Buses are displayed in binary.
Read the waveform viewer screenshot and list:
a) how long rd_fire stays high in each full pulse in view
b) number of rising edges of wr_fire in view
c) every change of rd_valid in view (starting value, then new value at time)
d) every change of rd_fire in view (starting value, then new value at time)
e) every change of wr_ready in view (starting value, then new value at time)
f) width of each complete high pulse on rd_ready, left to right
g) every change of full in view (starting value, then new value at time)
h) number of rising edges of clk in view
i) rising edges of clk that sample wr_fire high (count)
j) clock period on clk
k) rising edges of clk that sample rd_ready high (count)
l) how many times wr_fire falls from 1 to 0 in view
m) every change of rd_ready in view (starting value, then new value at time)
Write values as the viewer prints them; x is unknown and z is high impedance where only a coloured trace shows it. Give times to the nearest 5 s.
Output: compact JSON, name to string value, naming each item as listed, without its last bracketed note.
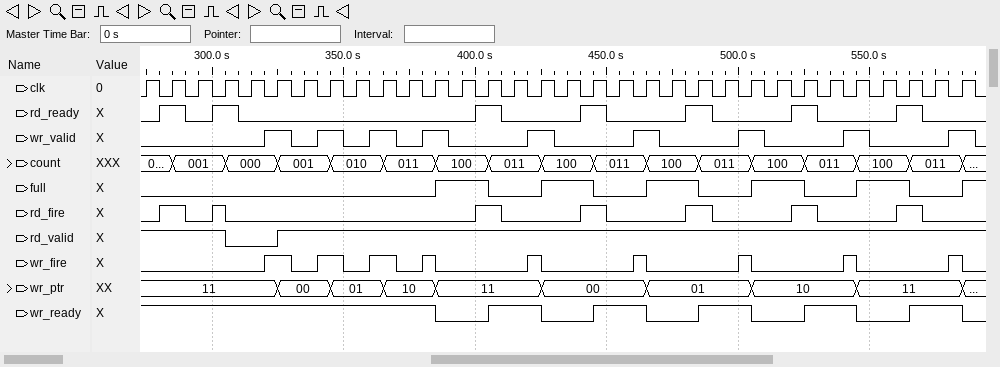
{"how long rd_fire stays high in each full pulse in view": "10 s, 5 s, 10 s, 10 s, 10 s, 10 s, 10 s", "number of rising edges of wr_fire in view": "9", "every change of rd_valid in view": "1, 0 at 305 s, 1 at 325 s", "every change of rd_fire in view": "0, 1 at 280 s, 0 at 290 s, 1 at 300 s, 0 at 305 s, 1 at 400 s, 0 at 410 s, 1 at 440 s, 0 at 450 s, 1 at 480 s, 0 at 490 s, 1 at 520 s, 0 at 530 s, 1 at 560 s, 0 at 570 s", "every change of wr_ready in view": "1, 0 at 385 s, 1 at 405 s, 0 at 425 s, 1 at 445 s, 0 at 465 s, 1 at 485 s, 0 at 505 s, 1 at 525 s, 0 at 545 s, 1 at 565 s, 0 at 585 s", "width of each complete high pulse on rd_ready, left to right": "10 s, 10 s, 10 s, 10 s, 10 s, 10 s, 10 s", "every change of full in view": "0, 1 at 385 s, 0 at 405 s, 1 at 425 s, 0 at 445 s, 1 at 465 s, 0 at 485 s, 1 at 505 s, 0 at 525 s, 1 at 545 s, 0 at 565 s, 1 at 585 s", "number of rising edges of clk in view": "32", "rising edges of clk that sample wr_fire high": "9", "clock period on clk": "10 s", "rising edges of clk that sample rd_ready high": "7", "how many times wr_fire falls from 1 to 0 in view": "9", "every change of rd_ready in view": "0, 1 at 280 s, 0 at 290 s, 1 at 300 s, 0 at 310 s, 1 at 400 s, 0 at 410 s, 1 at 440 s, 0 at 450 s, 1 at 480 s, 0 at 490 s, 1 at 520 s, 0 at 530 s, 1 at 560 s, 0 at 570 s"}
